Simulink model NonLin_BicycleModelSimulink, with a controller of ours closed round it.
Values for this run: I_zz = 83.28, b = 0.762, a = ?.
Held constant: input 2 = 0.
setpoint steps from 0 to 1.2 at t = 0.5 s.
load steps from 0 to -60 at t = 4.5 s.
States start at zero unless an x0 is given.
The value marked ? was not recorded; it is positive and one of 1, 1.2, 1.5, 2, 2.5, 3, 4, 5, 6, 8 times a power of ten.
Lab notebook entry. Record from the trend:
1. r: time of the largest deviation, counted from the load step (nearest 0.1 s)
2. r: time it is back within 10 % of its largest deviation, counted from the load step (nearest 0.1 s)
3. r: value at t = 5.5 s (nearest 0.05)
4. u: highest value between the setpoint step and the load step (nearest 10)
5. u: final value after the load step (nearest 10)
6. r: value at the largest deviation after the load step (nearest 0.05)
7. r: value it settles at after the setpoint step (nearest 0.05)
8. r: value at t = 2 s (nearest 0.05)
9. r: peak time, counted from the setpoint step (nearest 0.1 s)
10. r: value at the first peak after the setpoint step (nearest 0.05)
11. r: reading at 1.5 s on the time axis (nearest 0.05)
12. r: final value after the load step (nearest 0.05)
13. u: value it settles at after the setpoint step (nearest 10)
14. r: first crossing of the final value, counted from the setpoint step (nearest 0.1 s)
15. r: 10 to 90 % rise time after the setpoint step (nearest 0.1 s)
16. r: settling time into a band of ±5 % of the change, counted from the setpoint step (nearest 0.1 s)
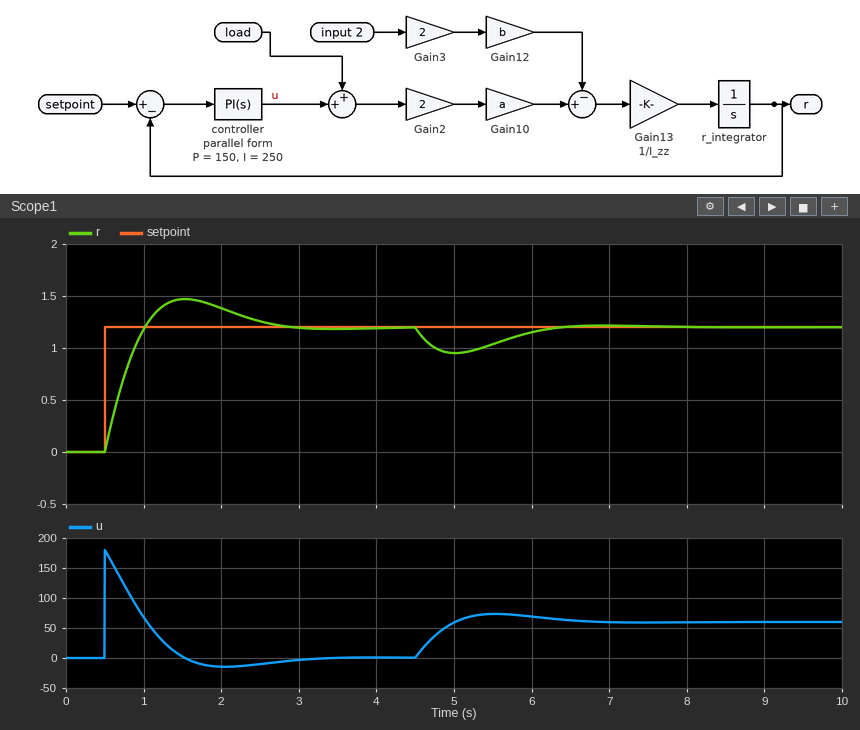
0.5 s
1.7 s
1.05
180
60
0.95
1.20
1.40
1.0 s
1.45
1.45
1.20
0
0.5 s
0.4 s
2.0 s
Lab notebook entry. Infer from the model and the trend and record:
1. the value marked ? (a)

0.8
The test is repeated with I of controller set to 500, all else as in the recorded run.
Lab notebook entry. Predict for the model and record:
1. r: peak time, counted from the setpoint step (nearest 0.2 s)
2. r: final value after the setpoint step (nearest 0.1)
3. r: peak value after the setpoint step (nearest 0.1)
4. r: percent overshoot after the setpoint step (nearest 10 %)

0.8 s
1.2
1.6
30 %
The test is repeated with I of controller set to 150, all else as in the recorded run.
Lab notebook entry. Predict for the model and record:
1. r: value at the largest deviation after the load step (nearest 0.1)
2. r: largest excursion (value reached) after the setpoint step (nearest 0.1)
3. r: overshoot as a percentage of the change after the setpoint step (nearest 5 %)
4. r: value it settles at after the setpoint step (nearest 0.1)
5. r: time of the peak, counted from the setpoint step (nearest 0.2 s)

0.9
1.4
15 %
1.2
1.2 s
